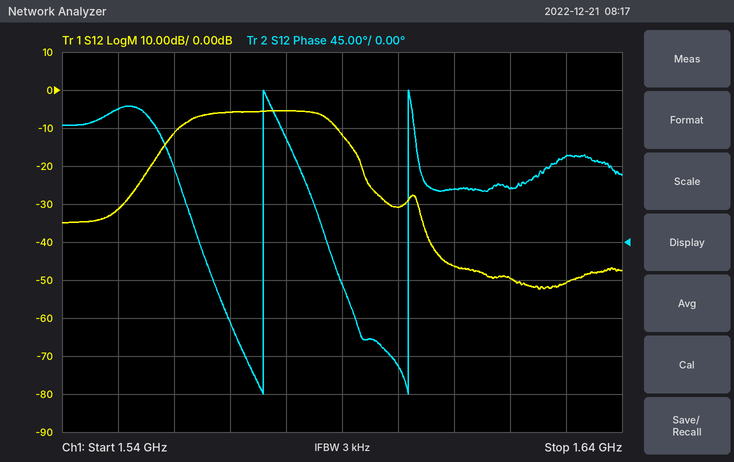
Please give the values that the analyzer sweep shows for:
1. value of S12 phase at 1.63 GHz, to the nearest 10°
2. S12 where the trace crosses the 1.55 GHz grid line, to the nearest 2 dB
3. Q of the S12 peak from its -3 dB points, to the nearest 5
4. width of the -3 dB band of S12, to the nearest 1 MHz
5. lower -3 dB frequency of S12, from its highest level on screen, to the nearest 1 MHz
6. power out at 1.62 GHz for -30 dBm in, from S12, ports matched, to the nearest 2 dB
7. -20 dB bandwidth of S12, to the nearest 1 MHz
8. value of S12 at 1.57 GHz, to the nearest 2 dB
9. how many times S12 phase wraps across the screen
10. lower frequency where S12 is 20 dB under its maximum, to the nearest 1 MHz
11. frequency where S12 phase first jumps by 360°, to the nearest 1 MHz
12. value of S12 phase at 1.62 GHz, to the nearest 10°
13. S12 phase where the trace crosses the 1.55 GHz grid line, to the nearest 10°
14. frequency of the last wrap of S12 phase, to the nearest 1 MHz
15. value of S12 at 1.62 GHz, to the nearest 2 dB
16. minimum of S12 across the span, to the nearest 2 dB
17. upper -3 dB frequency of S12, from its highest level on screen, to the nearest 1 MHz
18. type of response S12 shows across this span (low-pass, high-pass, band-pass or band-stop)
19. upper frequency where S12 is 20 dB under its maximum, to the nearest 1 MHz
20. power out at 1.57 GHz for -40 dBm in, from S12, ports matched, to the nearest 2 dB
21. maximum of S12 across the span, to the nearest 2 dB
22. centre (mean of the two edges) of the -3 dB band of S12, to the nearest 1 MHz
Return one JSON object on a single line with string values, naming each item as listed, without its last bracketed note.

{"value of S12 phase at 1.63 GHz, to the nearest 10°": "100°", "S12 where the trace crosses the 1.55 GHz grid line, to the nearest 2 dB": "-32 dB", "Q of the S12 peak from its -3 dB points, to the nearest 5": "60", "width of the -3 dB band of S12, to the nearest 1 MHz": "26 MHz", "lower -3 dB frequency of S12, from its highest level on screen, to the nearest 1 MHz": "1.562 GHz", "power out at 1.62 GHz for -30 dBm in, from S12, ports matched, to the nearest 2 dB": "-80 dBm", "-20 dB bandwidth of S12, to the nearest 1 MHz": "42 MHz", "value of S12 at 1.57 GHz, to the nearest 2 dB": "-6 dB", "how many times S12 phase wraps across the screen": "2", "lower frequency where S12 is 20 dB under its maximum, to the nearest 1 MHz": "1.553 GHz", "frequency where S12 phase first jumps by 360°, to the nearest 1 MHz": "1.576 GHz", "value of S12 phase at 1.62 GHz, to the nearest 10°": "60°", "S12 phase where the trace crosses the 1.55 GHz grid line, to the nearest 10°": "160°", "frequency of the last wrap of S12 phase, to the nearest 1 MHz": "1.602 GHz", "value of S12 at 1.62 GHz, to the nearest 2 dB": "-50 dB", "minimum of S12 across the span, to the nearest 2 dB": "-52 dB", "upper -3 dB frequency of S12, from its highest level on screen, to the nearest 1 MHz": "1.588 GHz", "type of response S12 shows across this span": "band-pass", "upper frequency where S12 is 20 dB under its maximum, to the nearest 1 MHz": "1.595 GHz", "power out at 1.57 GHz for -40 dBm in, from S12, ports matched, to the nearest 2 dB": "-46 dBm", "maximum of S12 across the span, to the nearest 2 dB": "-6 dB", "centre (mean of the two edges) of the -3 dB band of S12, to the nearest 1 MHz": "1.575 GHz"}
